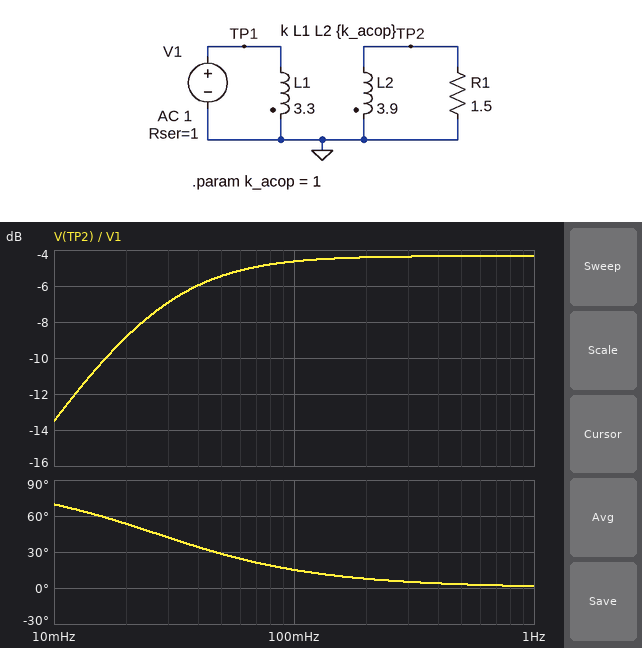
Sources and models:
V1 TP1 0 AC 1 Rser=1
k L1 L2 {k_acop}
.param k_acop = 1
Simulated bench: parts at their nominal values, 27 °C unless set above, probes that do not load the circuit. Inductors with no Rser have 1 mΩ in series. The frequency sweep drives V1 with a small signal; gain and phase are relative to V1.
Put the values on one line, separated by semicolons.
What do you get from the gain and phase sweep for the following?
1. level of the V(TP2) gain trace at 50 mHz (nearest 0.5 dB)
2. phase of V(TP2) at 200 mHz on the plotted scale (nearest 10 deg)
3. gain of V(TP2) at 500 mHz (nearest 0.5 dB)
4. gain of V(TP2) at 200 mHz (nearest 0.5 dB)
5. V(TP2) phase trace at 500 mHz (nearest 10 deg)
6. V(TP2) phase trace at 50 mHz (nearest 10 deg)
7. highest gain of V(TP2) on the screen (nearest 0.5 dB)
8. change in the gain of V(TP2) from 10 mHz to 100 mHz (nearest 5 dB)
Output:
-5.5 dB; 10 deg; -4.5 dB; -4.5 dB; 0 deg; 30 deg; -4.5 dB; 10 dB
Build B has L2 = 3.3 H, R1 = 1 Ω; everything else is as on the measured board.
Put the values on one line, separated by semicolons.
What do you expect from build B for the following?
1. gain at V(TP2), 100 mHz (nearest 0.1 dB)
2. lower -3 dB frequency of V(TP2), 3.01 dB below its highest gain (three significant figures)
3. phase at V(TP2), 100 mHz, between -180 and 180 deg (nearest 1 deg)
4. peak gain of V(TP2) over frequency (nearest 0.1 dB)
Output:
-6.3 dB; 24.1 mHz; 14 deg; -6.0 dB
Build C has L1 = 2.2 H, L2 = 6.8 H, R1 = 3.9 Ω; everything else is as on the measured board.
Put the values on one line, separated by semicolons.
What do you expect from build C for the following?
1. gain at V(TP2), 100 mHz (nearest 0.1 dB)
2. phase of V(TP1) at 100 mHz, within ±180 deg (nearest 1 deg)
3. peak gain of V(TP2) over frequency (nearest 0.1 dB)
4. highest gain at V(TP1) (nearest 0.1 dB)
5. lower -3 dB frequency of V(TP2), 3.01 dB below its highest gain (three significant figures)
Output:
-0.8 dB; 22 deg; -0.2 dB; -5.1 dB; 40.4 mHz
